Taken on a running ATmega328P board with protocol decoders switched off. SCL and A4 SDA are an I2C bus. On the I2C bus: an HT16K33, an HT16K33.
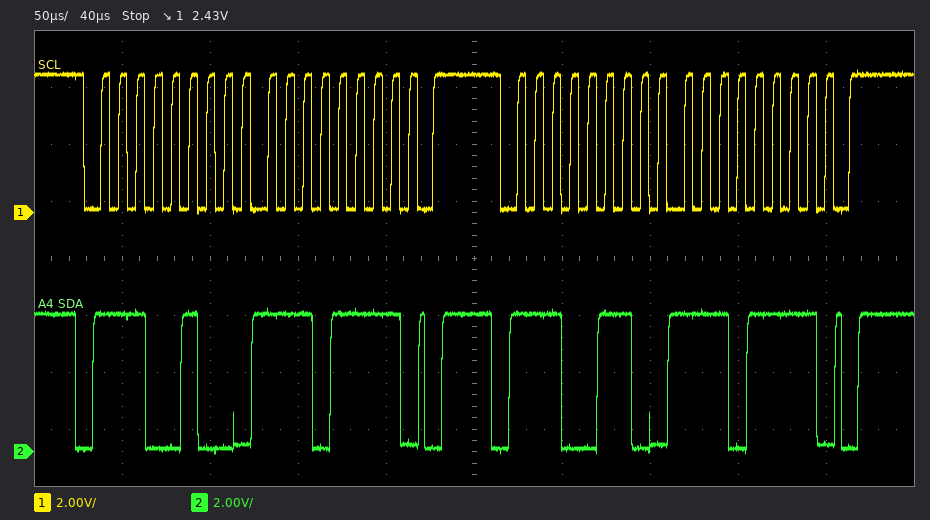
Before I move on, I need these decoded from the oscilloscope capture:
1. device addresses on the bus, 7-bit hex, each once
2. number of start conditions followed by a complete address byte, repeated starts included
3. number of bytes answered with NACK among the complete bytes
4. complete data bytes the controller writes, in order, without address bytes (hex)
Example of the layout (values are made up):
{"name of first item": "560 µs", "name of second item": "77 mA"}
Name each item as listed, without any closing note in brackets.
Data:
{"device addresses on the bus, 7-bit hex, each once": "0x72 0x73", "number of start conditions followed by a complete address byte, repeated starts included": "2", "number of bytes answered with NACK among the complete bytes": "0", "complete data bytes the controller writes, in order, without address bytes": "EF EF"}
